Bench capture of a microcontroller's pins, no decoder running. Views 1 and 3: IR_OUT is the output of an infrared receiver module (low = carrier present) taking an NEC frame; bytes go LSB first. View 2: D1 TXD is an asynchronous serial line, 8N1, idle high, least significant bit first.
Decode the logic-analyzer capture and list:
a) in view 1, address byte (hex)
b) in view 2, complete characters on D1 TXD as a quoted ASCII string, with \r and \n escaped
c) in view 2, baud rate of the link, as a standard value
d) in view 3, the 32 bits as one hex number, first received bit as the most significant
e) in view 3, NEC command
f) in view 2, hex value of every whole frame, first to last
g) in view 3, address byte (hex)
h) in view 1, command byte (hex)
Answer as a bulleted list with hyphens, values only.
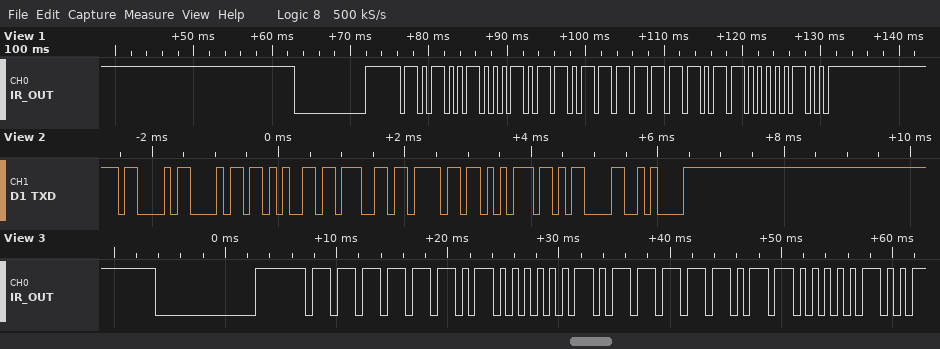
- 0x25
- "Chegou\r\n"
- 9600 baud
- 0xFD02FB04
- 0xDF
- 43 68 65 67 6F 75 0D 0A
- 0xBF
- 0xDF
